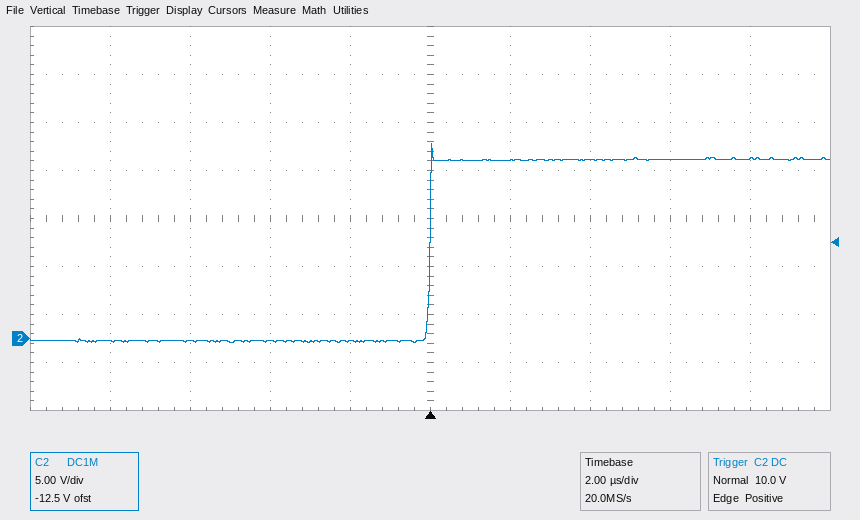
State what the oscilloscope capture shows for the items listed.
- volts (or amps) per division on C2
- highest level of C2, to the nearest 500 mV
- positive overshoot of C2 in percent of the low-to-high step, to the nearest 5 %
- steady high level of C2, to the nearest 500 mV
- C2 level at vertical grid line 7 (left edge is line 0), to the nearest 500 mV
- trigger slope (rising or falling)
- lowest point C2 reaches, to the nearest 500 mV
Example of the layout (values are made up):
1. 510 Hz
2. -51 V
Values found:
1. 5 V
2. 20.5 V
3. 10 %
4. 18.5 V
5. 18.5 V
6. rising
7. -500 mV
